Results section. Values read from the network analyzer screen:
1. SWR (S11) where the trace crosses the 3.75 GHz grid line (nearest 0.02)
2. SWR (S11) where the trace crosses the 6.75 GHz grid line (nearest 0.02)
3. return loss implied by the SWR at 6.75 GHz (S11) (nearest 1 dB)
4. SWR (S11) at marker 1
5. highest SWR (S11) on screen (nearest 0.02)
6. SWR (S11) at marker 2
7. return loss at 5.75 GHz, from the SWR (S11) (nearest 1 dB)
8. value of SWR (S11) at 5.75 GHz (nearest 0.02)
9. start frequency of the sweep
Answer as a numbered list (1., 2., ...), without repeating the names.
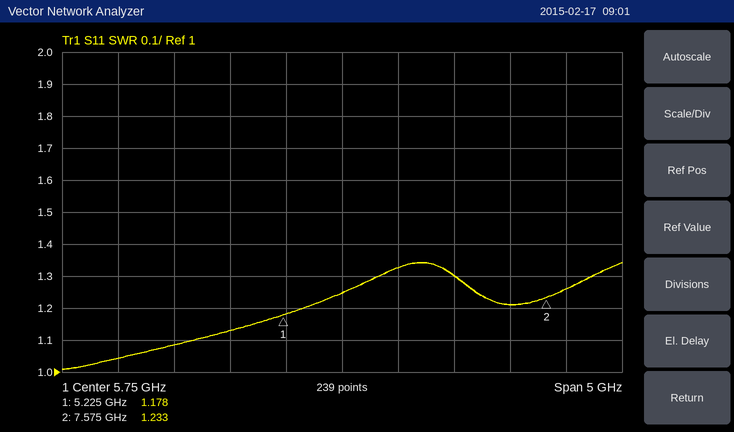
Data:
1. 1.04
2. 1.30
3. 18 dB
4. 1.178
5. 1.34
6. 1.233
7. 19 dB
8. 1.24
9. 3.25 GHz
